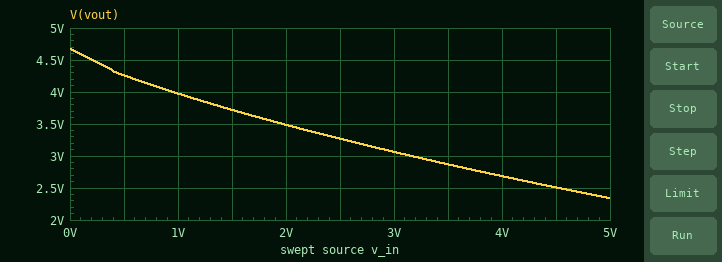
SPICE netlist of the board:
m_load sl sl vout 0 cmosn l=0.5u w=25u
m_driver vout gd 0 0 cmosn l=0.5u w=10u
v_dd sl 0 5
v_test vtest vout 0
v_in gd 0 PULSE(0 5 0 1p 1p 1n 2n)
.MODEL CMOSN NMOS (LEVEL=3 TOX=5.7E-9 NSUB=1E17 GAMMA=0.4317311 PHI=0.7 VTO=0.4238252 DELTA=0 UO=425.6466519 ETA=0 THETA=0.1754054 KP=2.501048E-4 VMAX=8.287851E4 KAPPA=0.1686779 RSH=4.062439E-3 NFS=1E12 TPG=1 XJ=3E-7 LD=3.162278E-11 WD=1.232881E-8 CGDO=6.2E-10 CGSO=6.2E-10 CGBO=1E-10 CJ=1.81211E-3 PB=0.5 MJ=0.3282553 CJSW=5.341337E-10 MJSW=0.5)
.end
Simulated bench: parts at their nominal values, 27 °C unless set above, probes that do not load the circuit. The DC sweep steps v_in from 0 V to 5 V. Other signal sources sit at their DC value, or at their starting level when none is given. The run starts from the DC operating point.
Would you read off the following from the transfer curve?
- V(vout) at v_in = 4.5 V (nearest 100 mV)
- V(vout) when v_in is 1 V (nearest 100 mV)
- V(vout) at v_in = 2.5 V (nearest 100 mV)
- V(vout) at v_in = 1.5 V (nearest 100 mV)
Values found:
2.5 V
4.0 V
3.3 V
3.7 V
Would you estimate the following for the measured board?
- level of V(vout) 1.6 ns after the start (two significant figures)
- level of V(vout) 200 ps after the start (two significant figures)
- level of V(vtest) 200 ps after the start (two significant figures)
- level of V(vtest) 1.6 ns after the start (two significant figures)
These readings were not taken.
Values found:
4.3 V
2.3 V
2.3 V
4.3 V
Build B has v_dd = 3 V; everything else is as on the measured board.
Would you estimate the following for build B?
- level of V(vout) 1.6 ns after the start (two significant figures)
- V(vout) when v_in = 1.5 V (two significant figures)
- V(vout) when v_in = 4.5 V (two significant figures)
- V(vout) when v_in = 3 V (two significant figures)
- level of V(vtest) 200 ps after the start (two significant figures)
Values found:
2.4 V
1.8 V
910 mV
1.2 V
850 mV
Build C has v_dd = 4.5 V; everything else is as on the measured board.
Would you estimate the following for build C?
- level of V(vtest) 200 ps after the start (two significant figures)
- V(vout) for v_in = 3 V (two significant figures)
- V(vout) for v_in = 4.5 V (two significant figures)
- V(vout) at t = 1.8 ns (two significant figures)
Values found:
1.9 V
2.6 V
2.1 V
3.9 V
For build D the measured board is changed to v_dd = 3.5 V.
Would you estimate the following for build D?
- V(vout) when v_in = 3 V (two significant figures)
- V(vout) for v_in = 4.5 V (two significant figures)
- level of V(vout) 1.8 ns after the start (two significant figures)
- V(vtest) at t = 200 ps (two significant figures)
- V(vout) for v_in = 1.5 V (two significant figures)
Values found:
1.7 V
1.2 V
2.9 V
1.1 V
2.3 V
